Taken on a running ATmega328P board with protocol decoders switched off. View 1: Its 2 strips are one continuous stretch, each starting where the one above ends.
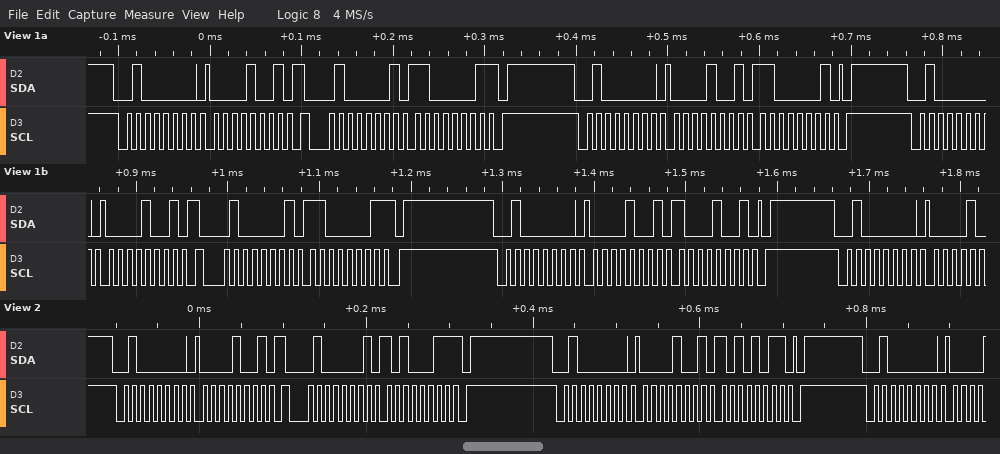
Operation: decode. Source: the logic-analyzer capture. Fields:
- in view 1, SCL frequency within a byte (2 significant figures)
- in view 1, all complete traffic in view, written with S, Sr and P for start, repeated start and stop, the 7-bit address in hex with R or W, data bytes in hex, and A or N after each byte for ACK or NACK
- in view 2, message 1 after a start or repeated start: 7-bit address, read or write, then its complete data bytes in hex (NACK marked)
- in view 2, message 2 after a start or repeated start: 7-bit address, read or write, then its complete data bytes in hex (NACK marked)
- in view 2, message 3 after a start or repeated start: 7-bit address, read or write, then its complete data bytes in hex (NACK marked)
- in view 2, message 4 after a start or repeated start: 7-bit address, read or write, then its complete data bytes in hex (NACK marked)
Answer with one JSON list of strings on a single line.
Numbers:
["100 kHz", "S 20W A 09 A Sr 20R A C1 N P S 20W A 09 A C1 A P S 20W A 09 A Sr 20R A C1 N P S 20W A 09 A 89 A P S 20W A", "0x20 write: 09", "0x20 read: A3 NACK", "0x20 write: 09 AB", "0x20 write"]
